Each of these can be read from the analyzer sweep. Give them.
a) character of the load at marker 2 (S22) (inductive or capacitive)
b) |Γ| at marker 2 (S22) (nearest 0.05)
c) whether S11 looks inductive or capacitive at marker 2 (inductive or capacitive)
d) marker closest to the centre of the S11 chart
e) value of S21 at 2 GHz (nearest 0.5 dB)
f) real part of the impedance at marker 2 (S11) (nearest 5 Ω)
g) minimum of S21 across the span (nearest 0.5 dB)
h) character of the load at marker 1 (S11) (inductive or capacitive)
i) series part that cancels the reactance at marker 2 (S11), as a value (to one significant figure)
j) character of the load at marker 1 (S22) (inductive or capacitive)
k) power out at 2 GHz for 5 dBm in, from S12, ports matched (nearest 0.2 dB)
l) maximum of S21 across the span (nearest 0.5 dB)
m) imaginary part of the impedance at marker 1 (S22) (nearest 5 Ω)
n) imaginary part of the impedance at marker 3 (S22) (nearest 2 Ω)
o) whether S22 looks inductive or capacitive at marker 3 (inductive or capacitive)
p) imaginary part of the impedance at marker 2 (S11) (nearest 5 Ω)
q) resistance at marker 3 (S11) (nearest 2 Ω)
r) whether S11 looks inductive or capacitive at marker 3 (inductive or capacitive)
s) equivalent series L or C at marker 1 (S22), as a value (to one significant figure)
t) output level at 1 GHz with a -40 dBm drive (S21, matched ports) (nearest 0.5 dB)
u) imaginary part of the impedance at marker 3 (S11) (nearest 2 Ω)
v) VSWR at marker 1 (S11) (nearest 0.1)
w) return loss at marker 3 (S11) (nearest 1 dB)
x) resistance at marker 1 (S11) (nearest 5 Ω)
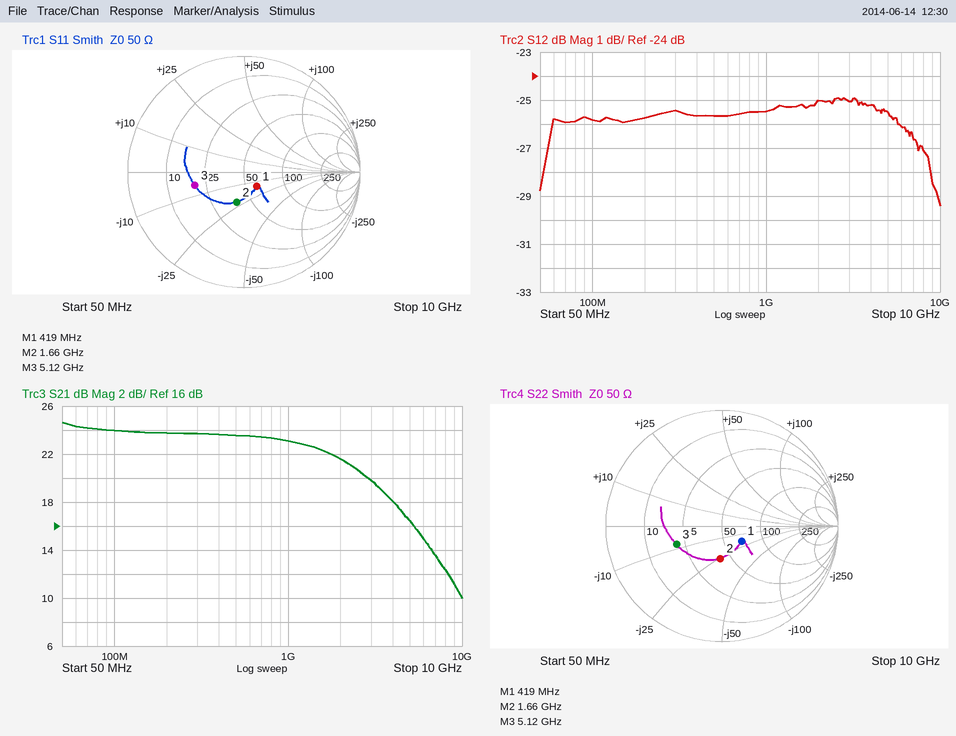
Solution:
capacitive
0.30
capacitive
marker 1
21.5 dB
40 Ω
10.0 dB
capacitive
2 nH
capacitive
-20.0 dBm
24.5 dB
-20 Ω
-8 Ω
capacitive
-20 Ω
20 Ω
capacitive
20 pF
-17.0 dBm
-6 Ω
1.4
7 dB
60 Ω
